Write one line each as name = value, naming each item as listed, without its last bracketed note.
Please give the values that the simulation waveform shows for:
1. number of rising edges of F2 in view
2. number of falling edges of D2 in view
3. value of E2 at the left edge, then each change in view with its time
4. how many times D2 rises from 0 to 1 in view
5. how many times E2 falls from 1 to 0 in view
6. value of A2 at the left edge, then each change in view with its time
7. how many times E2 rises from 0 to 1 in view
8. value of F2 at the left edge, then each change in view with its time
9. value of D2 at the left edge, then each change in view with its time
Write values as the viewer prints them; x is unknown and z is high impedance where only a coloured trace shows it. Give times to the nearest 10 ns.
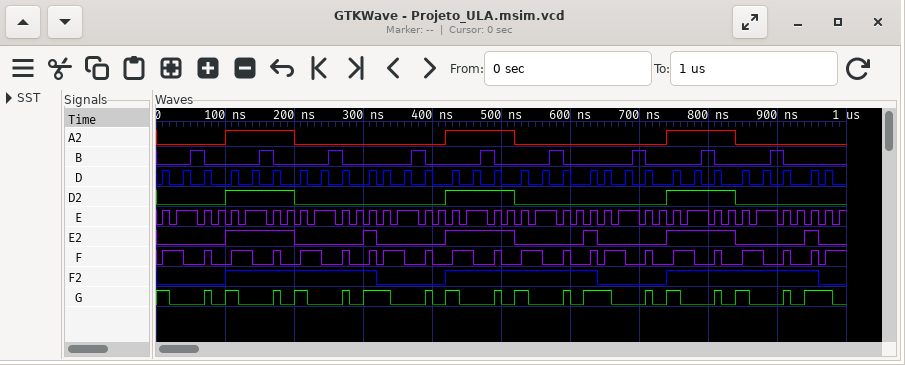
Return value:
number of rising edges of F2 in view = 3
number of falling edges of D2 in view = 3
value of E2 at the left edge, then each change in view with its time = 0, 1 at 100 ns, 0 at 200 ns, 1 at 300 ns, 0 at 320 ns, 1 at 420 ns, 0 at 520 ns, 1 at 620 ns, 0 at 640 ns, 1 at 740 ns, 0 at 840 ns, 1 at 940 ns, 0 at 960 ns
how many times D2 rises from 0 to 1 in view = 3
how many times E2 falls from 1 to 0 in view = 6
value of A2 at the left edge, then each change in view with its time = 0, 1 at 100 ns, 0 at 200 ns, 1 at 420 ns, 0 at 520 ns, 1 at 740 ns, 0 at 840 ns
how many times E2 rises from 0 to 1 in view = 6
value of F2 at the left edge, then each change in view with its time = 0, 1 at 100 ns, 0 at 320 ns, 1 at 420 ns, 0 at 640 ns, 1 at 740 ns, 0 at 960 ns
value of D2 at the left edge, then each change in view with its time = 0, 1 at 100 ns, 0 at 200 ns, 1 at 420 ns, 0 at 520 ns, 1 at 740 ns, 0 at 840 ns
